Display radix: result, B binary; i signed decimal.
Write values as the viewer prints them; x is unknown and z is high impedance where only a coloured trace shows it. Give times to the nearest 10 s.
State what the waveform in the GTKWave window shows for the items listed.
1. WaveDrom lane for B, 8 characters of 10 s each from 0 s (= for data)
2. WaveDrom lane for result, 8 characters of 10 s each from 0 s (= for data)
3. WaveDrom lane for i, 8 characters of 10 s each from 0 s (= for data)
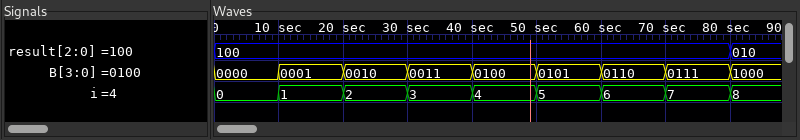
{name: 'B', wave: '========', data: '0000 0001 0010 0011 0100 0101 0110 0111'}
{name: 'result', wave: '=.......', data: '100'}
{name: 'i', wave: '========', data: '0 1 2 3 4 5 6 7'}
